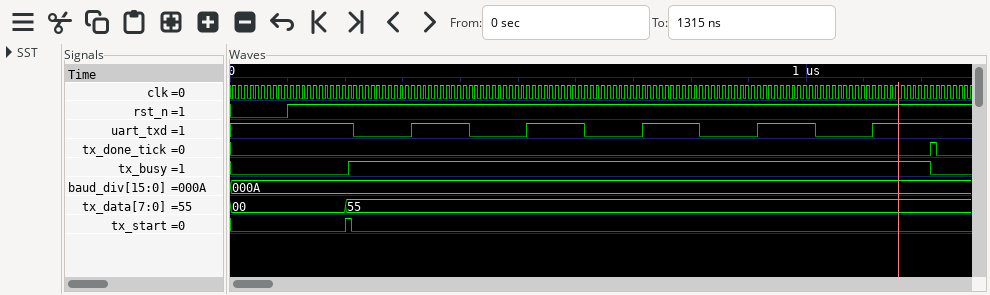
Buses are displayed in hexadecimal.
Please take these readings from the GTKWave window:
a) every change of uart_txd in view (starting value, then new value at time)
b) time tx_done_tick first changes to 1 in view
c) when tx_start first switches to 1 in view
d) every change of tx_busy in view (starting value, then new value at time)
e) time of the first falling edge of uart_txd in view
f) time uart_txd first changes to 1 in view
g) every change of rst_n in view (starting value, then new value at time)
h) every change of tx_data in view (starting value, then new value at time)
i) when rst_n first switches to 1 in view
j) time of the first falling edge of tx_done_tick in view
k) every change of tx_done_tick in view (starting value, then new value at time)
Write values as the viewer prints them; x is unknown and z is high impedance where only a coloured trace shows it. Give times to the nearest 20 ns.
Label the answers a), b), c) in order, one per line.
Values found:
a) 1, 0 at 220 ns, 1 at 320 ns, 0 at 420 ns, 1 at 520 ns, 0 at 620 ns, 1 at 720 ns, 0 at 820 ns, 1 at 920 ns, 0 at 1020 ns, 1 at 1120 ns
b) 1220 ns
c) 200 ns
d) 0, 1 at 200 ns, 0 at 1220 ns
e) 220 ns
f) 320 ns
g) 0, 1 at 100 ns
h) 00, 55 at 200 ns
i) 100 ns
j) 1220 ns
k) 0, 1 at 1220 ns, 0 at 1220 ns
